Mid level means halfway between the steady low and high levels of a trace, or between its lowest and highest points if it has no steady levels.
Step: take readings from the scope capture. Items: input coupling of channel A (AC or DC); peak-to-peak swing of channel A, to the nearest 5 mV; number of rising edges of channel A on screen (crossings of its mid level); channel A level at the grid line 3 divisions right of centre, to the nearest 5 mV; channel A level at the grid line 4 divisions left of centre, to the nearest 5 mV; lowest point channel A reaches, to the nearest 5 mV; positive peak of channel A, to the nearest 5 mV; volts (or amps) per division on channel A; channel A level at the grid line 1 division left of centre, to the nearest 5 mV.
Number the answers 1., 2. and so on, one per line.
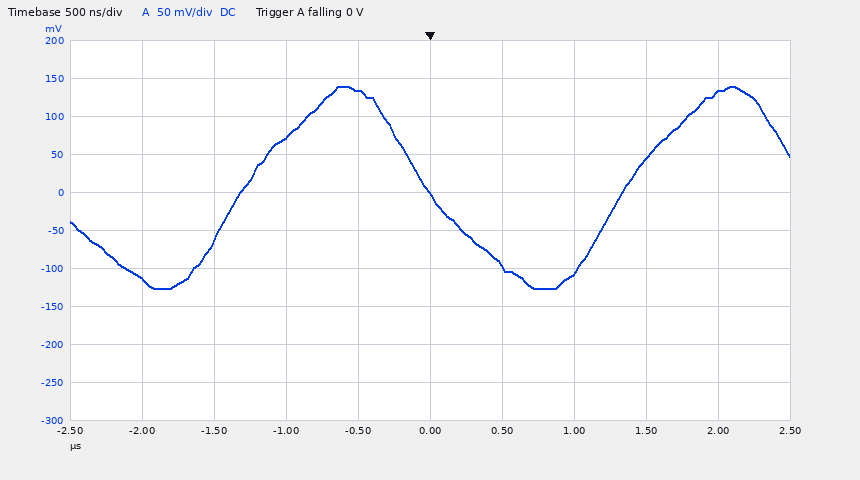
1. DC
2. 265 mV
3. 2
4. 45 mV
5. -115 mV
6. -125 mV
7. 140 mV
8. 50 mV
9. 135 mV
